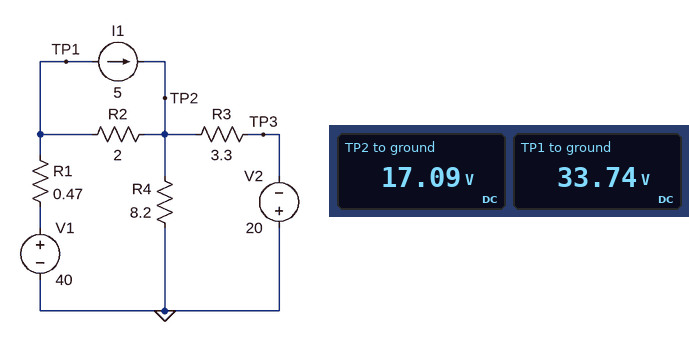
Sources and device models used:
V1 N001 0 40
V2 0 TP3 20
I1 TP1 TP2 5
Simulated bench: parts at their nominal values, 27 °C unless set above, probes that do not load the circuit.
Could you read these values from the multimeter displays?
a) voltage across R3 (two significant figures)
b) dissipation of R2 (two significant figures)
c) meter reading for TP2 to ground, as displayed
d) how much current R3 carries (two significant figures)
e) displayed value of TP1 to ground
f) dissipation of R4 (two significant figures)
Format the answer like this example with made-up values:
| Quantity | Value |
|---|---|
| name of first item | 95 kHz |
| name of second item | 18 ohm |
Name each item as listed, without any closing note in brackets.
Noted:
| Quantity | Value |
|---|---|
| voltage across R3 | 37 V |
| dissipation of R2 | 140 W |
| meter reading for TP2 to ground, as displayed | 17.09 V |
| how much current R3 carries | 11 A |
| displayed value of TP1 to ground | 33.74 V |
| dissipation of R4 | 36 W |
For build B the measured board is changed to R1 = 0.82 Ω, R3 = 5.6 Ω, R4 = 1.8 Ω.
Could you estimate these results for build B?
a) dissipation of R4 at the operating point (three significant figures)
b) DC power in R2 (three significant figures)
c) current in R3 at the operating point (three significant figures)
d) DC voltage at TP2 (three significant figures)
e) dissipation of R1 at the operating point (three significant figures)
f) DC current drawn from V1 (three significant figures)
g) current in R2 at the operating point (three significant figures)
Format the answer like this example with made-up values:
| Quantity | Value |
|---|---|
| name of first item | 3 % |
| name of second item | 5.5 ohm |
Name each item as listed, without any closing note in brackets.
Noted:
| Quantity | Value |
|---|---|
| dissipation of R4 at the operating point | 94.0 W |
| DC power in R2 | 132 W |
| current in R3 at the operating point | 5.89 A |
| DC voltage at TP2 | 13.0 V |
| dissipation of R1 at the operating point | 141 W |
| DC current drawn from V1 | 13.1 A |
| current in R2 at the operating point | 8.12 A |
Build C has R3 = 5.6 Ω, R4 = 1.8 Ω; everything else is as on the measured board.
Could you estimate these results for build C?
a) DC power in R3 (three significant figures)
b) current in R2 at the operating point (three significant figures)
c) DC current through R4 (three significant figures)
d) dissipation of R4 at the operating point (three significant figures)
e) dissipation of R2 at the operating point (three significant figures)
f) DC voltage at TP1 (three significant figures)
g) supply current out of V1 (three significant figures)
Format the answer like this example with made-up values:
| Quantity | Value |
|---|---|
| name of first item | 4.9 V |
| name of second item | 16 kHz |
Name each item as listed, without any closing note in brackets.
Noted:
| Quantity | Value |
|---|---|
| DC power in R3 | 214 W |
| current in R2 at the operating point | 9.32 A |
| DC current through R4 | 8.13 A |
| dissipation of R4 at the operating point | 119 W |
| dissipation of R2 at the operating point | 174 W |
| DC voltage at TP1 | 33.3 V |
| supply current out of V1 | 14.3 A |
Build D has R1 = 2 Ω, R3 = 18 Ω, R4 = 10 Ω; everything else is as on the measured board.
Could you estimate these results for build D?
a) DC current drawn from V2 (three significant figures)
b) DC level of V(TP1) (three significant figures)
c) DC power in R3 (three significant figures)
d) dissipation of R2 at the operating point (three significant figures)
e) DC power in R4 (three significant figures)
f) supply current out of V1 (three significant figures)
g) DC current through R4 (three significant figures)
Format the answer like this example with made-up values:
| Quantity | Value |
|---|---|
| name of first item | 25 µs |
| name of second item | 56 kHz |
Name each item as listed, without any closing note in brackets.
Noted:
| Quantity | Value |
|---|---|
| DC current drawn from V2 | 2.67 A |
| DC level of V(TP1) | 29.0 V |
| DC power in R3 | 128 W |
| dissipation of R2 at the operating point | 460 mW |
| DC power in R4 | 78.9 W |
| supply current out of V1 | 5.48 A |
| DC current through R4 | 2.81 A |
